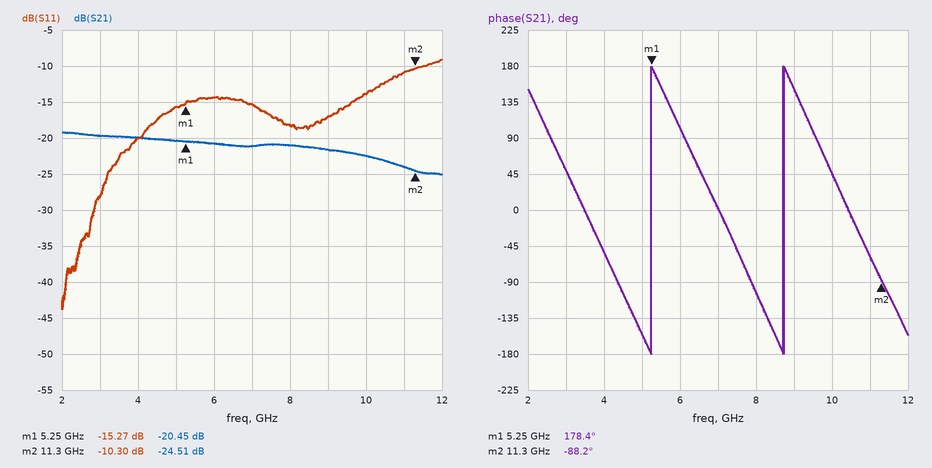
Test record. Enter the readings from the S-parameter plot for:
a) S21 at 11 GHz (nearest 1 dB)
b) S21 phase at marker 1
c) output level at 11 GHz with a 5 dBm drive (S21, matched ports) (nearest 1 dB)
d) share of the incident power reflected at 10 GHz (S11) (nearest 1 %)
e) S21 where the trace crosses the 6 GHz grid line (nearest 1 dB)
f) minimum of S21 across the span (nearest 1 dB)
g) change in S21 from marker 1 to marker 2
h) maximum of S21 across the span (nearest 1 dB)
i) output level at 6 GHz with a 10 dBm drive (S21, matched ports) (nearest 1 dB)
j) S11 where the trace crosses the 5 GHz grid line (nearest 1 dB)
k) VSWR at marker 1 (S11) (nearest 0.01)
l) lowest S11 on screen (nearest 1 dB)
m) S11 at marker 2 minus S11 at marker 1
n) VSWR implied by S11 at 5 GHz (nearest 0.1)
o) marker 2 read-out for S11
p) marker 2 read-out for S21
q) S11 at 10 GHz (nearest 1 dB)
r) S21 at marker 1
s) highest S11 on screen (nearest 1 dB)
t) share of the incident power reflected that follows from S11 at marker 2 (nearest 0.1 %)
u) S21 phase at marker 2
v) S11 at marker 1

-24 dB
178.4°
-19 dBm
4 %
-21 dB
-25 dB
-4.06 dB
-19 dB
-11 dBm
-16 dB
1.42
-44 dB
4.97 dB
1.4
-10.30 dB
-24.51 dB
-14 dB
-20.45 dB
-9 dB
9.3 %
-88.2°
-15.27 dB
